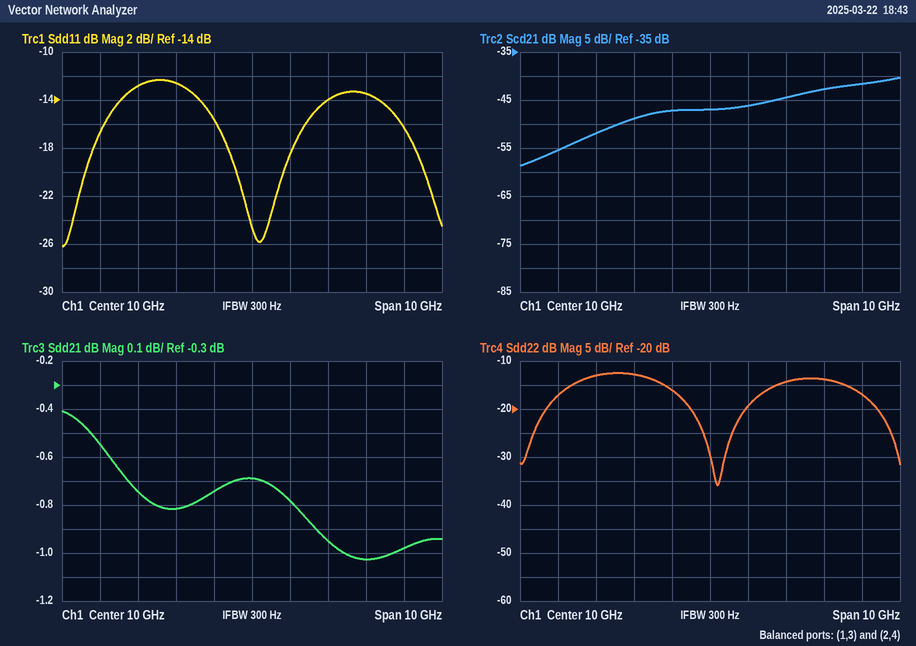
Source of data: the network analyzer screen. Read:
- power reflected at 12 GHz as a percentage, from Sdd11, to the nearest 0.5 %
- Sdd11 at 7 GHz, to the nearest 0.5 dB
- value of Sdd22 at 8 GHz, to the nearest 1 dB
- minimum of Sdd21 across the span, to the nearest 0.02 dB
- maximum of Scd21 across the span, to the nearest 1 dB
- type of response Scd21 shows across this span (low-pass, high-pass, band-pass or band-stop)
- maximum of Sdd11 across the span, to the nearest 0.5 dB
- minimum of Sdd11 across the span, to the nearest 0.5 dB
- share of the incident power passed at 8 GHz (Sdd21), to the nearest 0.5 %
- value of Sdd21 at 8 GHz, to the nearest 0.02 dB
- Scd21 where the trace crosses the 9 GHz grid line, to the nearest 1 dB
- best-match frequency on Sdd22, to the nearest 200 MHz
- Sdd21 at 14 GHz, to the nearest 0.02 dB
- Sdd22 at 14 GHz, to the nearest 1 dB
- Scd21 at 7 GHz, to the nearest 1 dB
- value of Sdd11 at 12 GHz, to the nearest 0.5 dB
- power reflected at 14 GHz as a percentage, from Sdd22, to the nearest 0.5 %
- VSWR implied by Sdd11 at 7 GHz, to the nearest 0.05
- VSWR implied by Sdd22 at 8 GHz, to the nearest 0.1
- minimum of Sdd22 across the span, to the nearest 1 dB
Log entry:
4.0 %
-13.0 dB
-13 dB
-1.02 dB
-40 dB
high-pass
-12.5 dB
-26.0 dB
83.0 %
-0.82 dB
-47 dB
10.2 GHz
-0.98 dB
-17 dB
-52 dB
-14.0 dB
2.0 %
1.60
1.6
-36 dB
